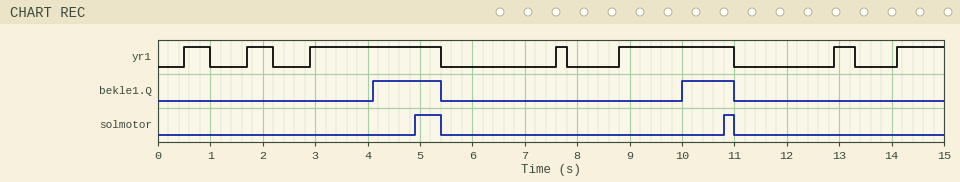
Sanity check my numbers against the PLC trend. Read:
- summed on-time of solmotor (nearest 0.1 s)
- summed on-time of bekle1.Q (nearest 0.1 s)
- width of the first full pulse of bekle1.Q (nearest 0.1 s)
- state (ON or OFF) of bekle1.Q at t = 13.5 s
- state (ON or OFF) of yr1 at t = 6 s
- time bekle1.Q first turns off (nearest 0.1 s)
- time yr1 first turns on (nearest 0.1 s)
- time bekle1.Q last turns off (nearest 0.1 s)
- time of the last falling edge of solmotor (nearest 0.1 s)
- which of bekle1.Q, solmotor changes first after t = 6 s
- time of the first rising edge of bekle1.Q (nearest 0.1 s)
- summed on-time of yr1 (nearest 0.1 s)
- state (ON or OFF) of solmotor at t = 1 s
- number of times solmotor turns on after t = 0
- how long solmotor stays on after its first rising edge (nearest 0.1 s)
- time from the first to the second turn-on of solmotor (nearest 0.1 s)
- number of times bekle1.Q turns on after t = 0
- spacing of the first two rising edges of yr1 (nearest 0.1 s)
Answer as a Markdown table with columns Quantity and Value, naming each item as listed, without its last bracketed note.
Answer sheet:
| Quantity | Value |
|---|---|
| summed on-time of solmotor | 0.7 s |
| summed on-time of bekle1.Q | 2.3 s |
| width of the first full pulse of bekle1.Q | 1.3 s |
| state (ON or OFF) of bekle1.Q at t = 13.5 s | OFF |
| state (ON or OFF) of yr1 at t = 6 s | OFF |
| time bekle1.Q first turns off | 5.4 s |
| time yr1 first turns on | 0.5 s |
| time bekle1.Q last turns off | 11.0 s |
| time of the last falling edge of solmotor | 11.0 s |
| which of bekle1.Q, solmotor changes first after t = 6 s | bekle1.Q |
| time of the first rising edge of bekle1.Q | 4.1 s |
| summed on-time of yr1 | 7.2 s |
| state (ON or OFF) of solmotor at t = 1 s | OFF |
| number of times solmotor turns on after t = 0 | 2 |
| how long solmotor stays on after its first rising edge | 0.5 s |
| time from the first to the second turn-on of solmotor | 5.9 s |
| number of times bekle1.Q turns on after t = 0 | 2 |
| spacing of the first two rising edges of yr1 | 1.2 s |
